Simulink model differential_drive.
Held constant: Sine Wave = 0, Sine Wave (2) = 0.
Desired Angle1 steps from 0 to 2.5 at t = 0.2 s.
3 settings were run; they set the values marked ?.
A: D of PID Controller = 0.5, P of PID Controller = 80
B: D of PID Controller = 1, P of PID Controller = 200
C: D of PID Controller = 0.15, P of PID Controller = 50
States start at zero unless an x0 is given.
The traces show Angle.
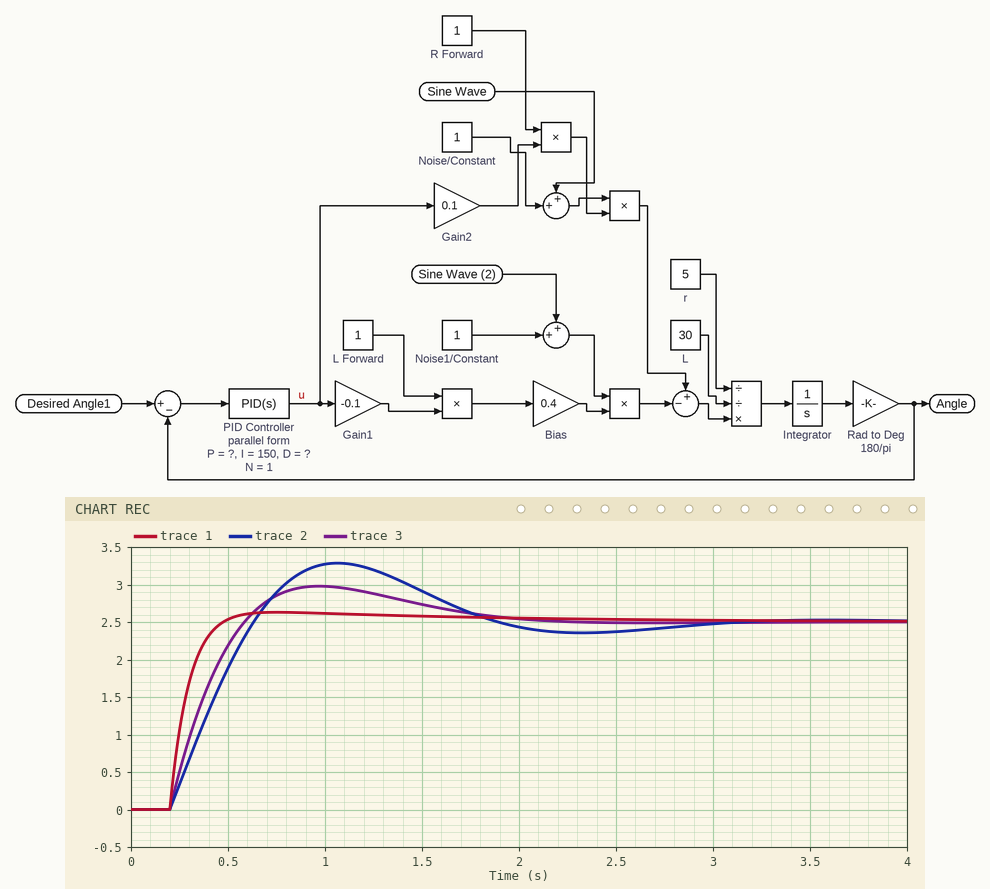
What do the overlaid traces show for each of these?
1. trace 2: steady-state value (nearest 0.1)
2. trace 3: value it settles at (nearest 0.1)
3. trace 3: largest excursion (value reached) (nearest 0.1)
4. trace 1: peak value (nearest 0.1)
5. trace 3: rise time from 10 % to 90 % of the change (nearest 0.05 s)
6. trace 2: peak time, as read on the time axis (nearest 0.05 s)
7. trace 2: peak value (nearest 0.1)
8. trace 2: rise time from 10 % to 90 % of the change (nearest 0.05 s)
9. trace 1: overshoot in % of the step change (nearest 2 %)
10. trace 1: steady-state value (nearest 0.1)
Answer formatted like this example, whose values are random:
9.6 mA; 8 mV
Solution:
2.5; 2.5; 3.0; 2.6; 0.30 s; 1.05 s; 3.3; 0.35 s; 6 %; 2.5
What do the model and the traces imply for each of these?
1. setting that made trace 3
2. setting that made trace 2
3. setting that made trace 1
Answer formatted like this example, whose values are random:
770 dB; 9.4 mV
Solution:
A; C; B
